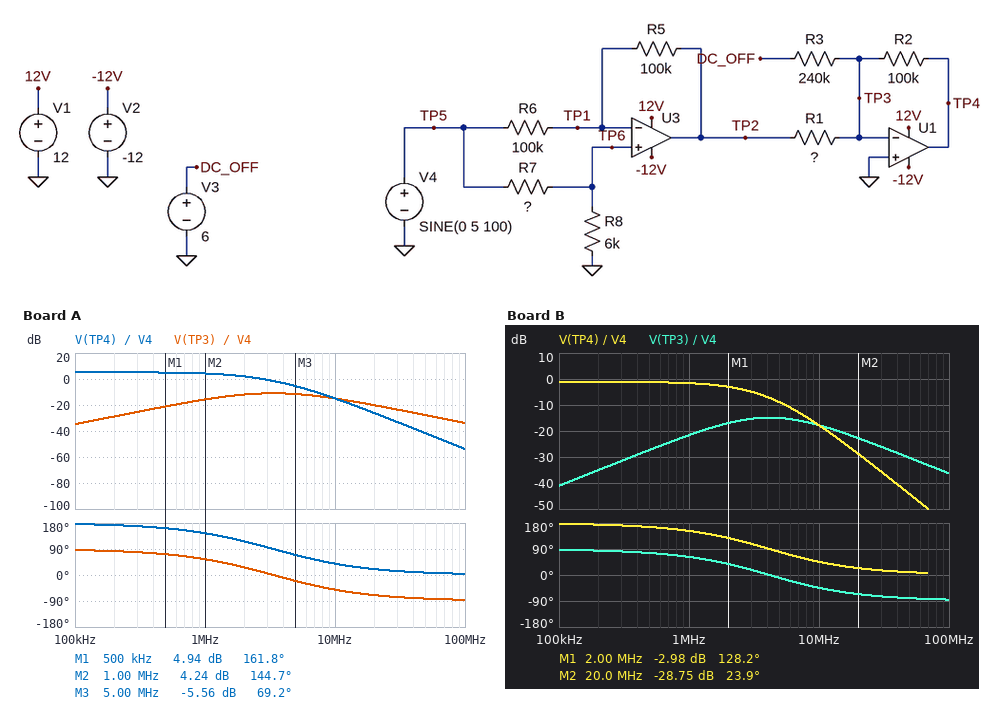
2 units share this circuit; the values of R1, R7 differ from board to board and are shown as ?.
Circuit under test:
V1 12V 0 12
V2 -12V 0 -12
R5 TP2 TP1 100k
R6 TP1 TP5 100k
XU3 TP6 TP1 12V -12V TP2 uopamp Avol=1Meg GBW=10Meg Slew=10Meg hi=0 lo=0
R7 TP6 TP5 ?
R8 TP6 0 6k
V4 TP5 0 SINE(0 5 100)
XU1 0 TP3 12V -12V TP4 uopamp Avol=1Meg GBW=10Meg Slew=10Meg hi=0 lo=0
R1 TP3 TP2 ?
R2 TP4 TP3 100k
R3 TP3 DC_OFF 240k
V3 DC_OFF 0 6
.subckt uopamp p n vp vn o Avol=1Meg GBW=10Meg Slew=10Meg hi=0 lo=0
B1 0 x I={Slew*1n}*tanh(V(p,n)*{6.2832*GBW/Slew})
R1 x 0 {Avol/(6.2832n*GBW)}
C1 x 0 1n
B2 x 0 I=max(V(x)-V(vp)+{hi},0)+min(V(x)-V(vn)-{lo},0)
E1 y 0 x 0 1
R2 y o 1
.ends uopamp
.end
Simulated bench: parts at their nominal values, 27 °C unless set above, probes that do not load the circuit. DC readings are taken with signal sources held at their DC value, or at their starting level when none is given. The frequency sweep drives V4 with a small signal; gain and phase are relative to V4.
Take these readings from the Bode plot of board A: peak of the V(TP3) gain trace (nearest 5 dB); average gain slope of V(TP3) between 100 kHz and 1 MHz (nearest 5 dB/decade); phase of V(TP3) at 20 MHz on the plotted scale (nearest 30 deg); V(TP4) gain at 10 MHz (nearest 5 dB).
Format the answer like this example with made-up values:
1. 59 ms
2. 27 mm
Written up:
1. -10 dB
2. 20 dB/decade
3. -60 deg
4. -15 dB
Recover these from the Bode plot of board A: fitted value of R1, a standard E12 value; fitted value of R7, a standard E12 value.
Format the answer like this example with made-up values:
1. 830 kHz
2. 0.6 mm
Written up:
1. 33 kΩ
2. 1.5 kΩ
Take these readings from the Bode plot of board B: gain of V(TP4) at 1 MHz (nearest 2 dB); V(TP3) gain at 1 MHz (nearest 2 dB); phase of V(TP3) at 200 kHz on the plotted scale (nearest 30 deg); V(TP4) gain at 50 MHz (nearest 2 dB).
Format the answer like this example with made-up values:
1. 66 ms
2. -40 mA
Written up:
1. -2 dB
2. -22 dB
3. 90 deg
4. -44 dB
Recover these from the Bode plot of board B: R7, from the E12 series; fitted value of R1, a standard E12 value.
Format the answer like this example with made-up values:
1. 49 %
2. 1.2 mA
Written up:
1. 1.5 kΩ
2. 68 kΩ
